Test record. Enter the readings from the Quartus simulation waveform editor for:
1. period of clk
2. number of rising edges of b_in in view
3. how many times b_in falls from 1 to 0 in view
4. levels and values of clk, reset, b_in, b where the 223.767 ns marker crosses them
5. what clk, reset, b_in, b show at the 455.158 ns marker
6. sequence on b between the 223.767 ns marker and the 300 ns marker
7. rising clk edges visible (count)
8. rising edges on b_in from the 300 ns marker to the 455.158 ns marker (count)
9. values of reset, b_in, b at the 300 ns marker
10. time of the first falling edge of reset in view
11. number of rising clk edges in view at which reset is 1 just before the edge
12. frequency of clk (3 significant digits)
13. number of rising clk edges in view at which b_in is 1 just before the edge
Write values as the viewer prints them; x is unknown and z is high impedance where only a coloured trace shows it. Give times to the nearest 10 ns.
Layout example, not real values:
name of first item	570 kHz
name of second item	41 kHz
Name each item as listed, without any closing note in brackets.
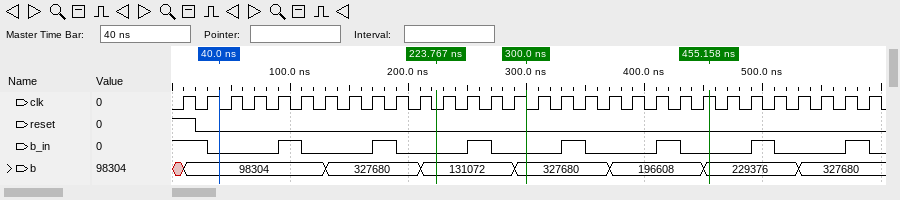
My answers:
period of clk	20 ns
number of rising edges of b_in in view	7
how many times b_in falls from 1 to 0 in view	8
levels and values of clk, reset, b_in, b where the 223.767 ns marker crosses them	clk=0, reset=0, b_in=0, b=131072
what clk, reset, b_in, b show at the 455.158 ns marker	clk=1, reset=0, b_in=0, b=229376
sequence on b between the 223.767 ns marker and the 300 ns marker	131072, 327680
rising clk edges visible	30
rising edges on b_in from the 300 ns marker to the 455.158 ns marker	2
values of reset, b_in, b at the 300 ns marker	reset=0, b_in=0, b=327680
time of the first falling edge of reset in view	20 ns
number of rising clk edges in view at which reset is 1 just before the edge	1
frequency of clk	50.0 MHz
number of rising clk edges in view at which b_in is 1 just before the edge	9
